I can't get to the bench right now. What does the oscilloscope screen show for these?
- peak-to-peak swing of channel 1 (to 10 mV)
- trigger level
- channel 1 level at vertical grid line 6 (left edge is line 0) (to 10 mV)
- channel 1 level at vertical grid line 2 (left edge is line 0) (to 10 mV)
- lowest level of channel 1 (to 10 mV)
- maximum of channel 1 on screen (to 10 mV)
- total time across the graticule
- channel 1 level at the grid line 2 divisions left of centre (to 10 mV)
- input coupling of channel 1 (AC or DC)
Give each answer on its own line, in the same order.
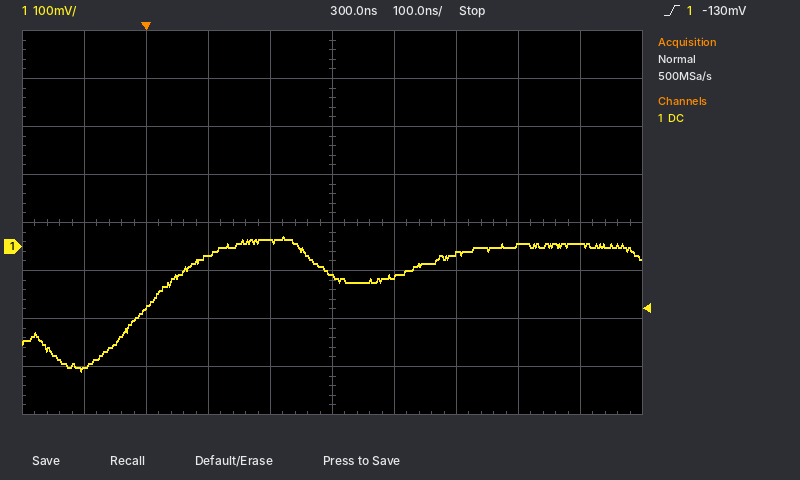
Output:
280 mV
-130 mV
-60 mV
-130 mV
-260 mV
20 mV
1 µs
-20 mV
DC
